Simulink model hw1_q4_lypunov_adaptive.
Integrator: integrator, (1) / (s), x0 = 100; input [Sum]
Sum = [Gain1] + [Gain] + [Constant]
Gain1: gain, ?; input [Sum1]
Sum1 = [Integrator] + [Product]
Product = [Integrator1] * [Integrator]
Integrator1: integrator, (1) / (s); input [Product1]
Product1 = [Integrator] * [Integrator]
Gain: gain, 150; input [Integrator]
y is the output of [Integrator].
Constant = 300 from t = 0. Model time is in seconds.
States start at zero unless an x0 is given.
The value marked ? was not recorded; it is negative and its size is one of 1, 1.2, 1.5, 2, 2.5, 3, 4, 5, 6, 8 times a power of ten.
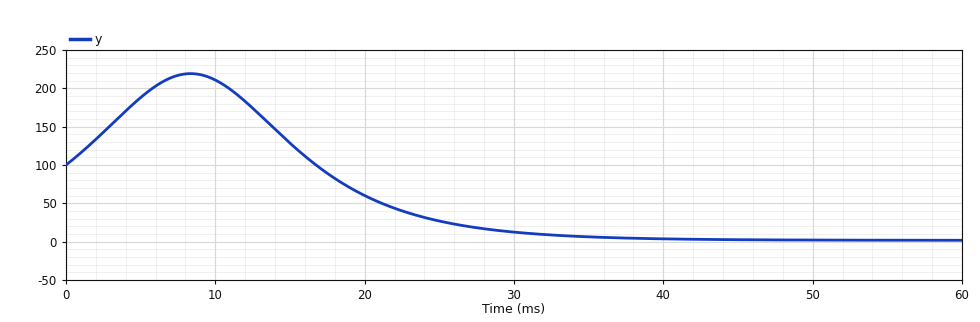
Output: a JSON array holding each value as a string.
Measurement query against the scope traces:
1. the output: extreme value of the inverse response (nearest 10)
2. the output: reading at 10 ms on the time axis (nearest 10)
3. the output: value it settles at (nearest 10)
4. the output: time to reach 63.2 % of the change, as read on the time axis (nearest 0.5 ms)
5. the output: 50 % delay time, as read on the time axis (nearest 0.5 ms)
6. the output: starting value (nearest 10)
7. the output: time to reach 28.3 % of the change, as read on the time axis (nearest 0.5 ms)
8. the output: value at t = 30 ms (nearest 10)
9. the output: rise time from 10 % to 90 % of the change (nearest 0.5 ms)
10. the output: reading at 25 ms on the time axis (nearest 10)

["220", "210", "0", "23.0 ms", "21.0 ms", "100", "19.0 ms", "10", "13.0 ms", "30"]
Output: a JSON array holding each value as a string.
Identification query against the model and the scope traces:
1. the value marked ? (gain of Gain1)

["-0.6"]
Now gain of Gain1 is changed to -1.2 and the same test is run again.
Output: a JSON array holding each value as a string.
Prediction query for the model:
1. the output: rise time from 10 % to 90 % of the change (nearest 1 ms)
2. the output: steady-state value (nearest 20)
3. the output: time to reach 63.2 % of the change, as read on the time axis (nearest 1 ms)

["12 ms", "0", "18 ms"]
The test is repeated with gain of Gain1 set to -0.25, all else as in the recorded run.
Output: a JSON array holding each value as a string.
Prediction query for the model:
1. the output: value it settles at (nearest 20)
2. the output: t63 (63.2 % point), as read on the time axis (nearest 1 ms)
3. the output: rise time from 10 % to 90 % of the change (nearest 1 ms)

["0", "29 ms", "14 ms"]
